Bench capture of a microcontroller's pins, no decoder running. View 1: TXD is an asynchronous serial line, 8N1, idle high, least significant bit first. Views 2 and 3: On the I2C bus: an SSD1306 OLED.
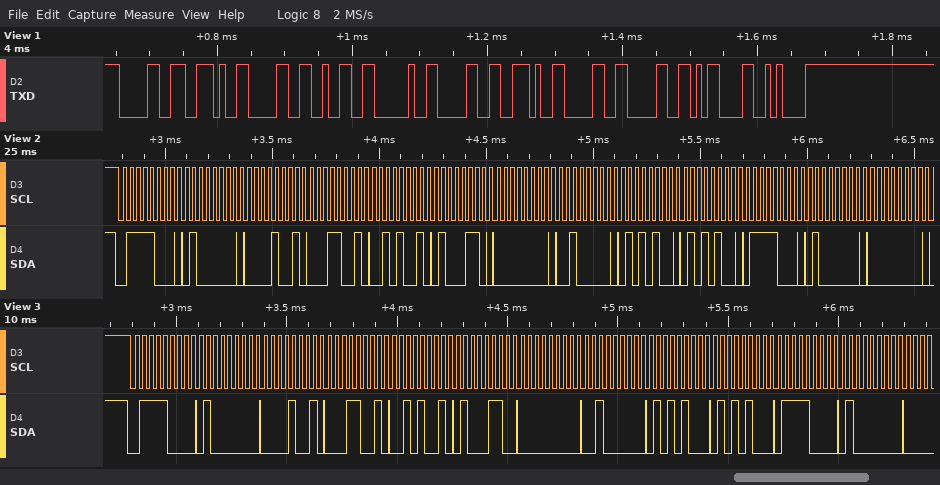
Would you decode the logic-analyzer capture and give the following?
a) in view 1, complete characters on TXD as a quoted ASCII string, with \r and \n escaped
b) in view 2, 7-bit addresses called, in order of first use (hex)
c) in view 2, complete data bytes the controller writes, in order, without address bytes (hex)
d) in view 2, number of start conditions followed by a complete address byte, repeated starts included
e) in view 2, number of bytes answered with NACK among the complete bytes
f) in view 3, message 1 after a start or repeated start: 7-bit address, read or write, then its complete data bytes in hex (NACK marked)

"0.02 0.00\r\n"
0x3C
40 09 19 29 46 00 20 54 54 78 40 00
1
0
0x3C write: 40 09 19 29 46 00 20 54 54 78 40
